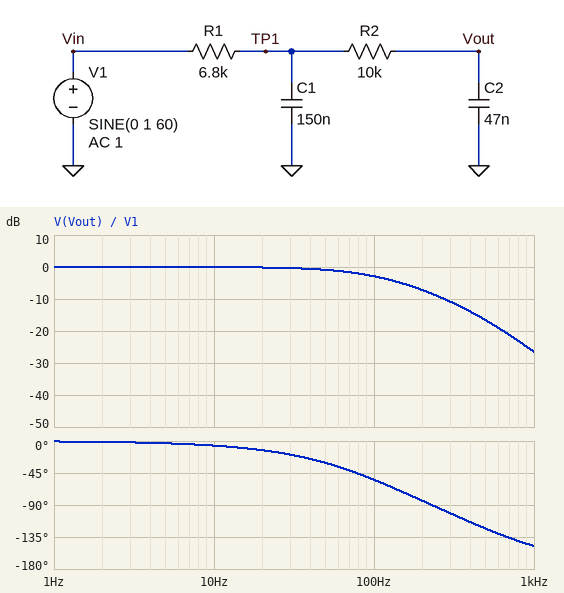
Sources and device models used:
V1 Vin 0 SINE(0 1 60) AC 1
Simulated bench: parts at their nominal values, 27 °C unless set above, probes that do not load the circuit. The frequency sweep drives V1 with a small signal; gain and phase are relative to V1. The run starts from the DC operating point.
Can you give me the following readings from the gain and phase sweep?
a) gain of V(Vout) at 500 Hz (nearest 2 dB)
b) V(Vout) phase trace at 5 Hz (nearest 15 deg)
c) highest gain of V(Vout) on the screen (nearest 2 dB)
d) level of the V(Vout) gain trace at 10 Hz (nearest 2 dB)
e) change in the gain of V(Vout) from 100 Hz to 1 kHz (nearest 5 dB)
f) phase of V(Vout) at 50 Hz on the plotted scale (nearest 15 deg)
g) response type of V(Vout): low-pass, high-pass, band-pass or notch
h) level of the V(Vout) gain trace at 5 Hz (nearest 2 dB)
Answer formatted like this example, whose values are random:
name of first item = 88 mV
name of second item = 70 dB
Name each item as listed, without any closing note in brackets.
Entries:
gain of V(Vout) at 500 Hz = -16 dB
V(Vout) phase trace at 5 Hz = 0 deg
highest gain of V(Vout) on the screen = 0 dB
level of the V(Vout) gain trace at 10 Hz = 0 dB
change in the gain of V(Vout) from 100 Hz to 1 kHz = -25 dB
phase of V(Vout) at 50 Hz on the plotted scale = -30 deg
response type of V(Vout): low-pass, high-pass, band-pass or notch = low-pass
level of the V(Vout) gain trace at 5 Hz = 0 dB
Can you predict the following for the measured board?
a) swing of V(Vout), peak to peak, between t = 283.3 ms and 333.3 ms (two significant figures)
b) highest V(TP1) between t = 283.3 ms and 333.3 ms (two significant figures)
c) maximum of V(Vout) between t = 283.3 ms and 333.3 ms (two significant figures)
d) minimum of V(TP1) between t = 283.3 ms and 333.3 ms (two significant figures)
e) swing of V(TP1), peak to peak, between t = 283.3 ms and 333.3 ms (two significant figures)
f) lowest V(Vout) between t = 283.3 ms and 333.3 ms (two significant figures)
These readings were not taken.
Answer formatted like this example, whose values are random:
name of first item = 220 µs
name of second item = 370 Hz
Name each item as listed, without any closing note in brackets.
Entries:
swing of V(Vout), peak to peak, between t = 283.3 ms and 333.3 ms = 1.7 V
highest V(TP1) between t = 283.3 ms and 333.3 ms = 880 mV
maximum of V(Vout) between t = 283.3 ms and 333.3 ms = 870 mV
minimum of V(TP1) between t = 283.3 ms and 333.3 ms = -880 mV
swing of V(TP1), peak to peak, between t = 283.3 ms and 333.3 ms = 1.8 V
lowest V(Vout) between t = 283.3 ms and 333.3 ms = -870 mV
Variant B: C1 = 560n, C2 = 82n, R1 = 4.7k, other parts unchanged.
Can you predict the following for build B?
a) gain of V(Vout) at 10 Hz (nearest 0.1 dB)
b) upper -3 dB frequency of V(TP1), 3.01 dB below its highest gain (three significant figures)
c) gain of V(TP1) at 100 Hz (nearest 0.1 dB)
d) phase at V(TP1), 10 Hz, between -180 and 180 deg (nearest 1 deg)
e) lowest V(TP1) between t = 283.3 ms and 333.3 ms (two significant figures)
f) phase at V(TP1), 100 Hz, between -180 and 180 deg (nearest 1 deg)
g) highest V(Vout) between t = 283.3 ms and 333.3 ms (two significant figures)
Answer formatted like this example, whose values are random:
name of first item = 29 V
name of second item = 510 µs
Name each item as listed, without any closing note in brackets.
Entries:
gain of V(Vout) at 10 Hz = -0.2 dB
upper -3 dB frequency of V(TP1), 3.01 dB below its highest gain = 51.5 Hz
gain of V(TP1) at 100 Hz = -6.6 dB
phase at V(TP1), 10 Hz, between -180 and 180 deg = -11 deg
lowest V(TP1) between t = 283.3 ms and 333.3 ms = -650 mV
phase at V(TP1), 100 Hz, between -180 and 180 deg = -59 deg
highest V(Vout) between t = 283.3 ms and 333.3 ms = 620 mV
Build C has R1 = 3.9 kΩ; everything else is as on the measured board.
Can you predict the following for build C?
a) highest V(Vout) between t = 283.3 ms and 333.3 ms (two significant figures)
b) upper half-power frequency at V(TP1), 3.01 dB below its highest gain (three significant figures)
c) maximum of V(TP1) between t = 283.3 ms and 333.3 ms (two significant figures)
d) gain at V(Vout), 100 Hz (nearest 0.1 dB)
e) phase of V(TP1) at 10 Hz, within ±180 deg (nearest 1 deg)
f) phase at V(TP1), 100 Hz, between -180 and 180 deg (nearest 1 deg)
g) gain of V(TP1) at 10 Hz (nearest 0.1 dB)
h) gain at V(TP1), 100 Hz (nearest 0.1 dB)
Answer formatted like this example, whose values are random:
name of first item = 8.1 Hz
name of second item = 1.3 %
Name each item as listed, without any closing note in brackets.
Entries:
highest V(Vout) between t = 283.3 ms and 333.3 ms = 940 mV
upper half-power frequency at V(TP1), 3.01 dB below its highest gain = 196 Hz
maximum of V(TP1) between t = 283.3 ms and 333.3 ms = 950 mV
gain at V(Vout), 100 Hz = -1.5 dB
phase of V(TP1) at 10 Hz, within ±180 deg = -3 deg
phase at V(TP1), 100 Hz, between -180 and 180 deg = -25 deg
gain of V(TP1) at 10 Hz = 0 dB
gain at V(TP1), 100 Hz = -1.1 dB
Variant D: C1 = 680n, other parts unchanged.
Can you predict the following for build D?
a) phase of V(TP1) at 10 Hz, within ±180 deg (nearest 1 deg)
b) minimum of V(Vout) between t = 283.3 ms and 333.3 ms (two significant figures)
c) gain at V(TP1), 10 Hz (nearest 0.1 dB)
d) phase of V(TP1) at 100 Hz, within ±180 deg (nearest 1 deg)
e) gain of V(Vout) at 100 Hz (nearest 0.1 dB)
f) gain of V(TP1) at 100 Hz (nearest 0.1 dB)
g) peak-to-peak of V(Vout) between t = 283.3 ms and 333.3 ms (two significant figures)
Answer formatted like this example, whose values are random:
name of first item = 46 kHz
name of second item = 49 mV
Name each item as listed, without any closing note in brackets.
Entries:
phase of V(TP1) at 10 Hz, within ±180 deg = -17 deg
minimum of V(Vout) between t = 283.3 ms and 333.3 ms = -460 mV
gain at V(TP1), 10 Hz = -0.4 dB
phase of V(TP1) at 100 Hz, within ±180 deg = -71 deg
gain of V(Vout) at 100 Hz = -10.6 dB
gain of V(TP1) at 100 Hz = -10.3 dB
peak-to-peak of V(Vout) between t = 283.3 ms and 333.3 ms = 930 mV
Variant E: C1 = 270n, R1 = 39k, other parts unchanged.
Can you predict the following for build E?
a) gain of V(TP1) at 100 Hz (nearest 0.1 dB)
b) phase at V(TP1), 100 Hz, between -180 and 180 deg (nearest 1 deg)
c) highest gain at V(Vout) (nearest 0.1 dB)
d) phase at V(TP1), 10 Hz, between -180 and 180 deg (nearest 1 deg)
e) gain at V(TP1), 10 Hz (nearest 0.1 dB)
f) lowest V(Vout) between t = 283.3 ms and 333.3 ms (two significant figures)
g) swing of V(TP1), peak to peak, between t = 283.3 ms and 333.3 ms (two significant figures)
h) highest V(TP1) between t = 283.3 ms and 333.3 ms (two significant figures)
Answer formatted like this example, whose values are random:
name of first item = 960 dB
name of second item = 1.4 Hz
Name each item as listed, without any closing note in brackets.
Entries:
gain of V(TP1) at 100 Hz = -17.8 dB
phase at V(TP1), 100 Hz, between -180 and 180 deg = -80 deg
highest gain at V(Vout) = 0 dB
phase at V(TP1), 10 Hz, between -180 and 180 deg = -38 deg
gain at V(TP1), 10 Hz = -2.1 dB
lowest V(Vout) between t = 283.3 ms and 333.3 ms = -210 mV
swing of V(TP1), peak to peak, between t = 283.3 ms and 333.3 ms = 420 mV
highest V(TP1) between t = 283.3 ms and 333.3 ms = 210 mV
